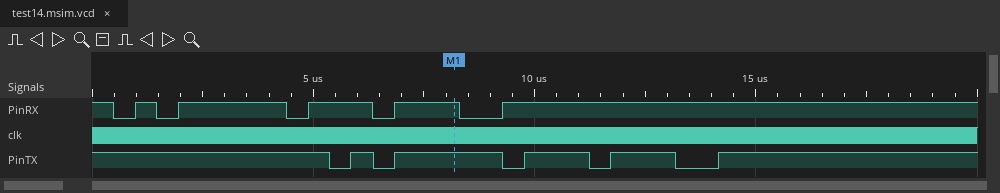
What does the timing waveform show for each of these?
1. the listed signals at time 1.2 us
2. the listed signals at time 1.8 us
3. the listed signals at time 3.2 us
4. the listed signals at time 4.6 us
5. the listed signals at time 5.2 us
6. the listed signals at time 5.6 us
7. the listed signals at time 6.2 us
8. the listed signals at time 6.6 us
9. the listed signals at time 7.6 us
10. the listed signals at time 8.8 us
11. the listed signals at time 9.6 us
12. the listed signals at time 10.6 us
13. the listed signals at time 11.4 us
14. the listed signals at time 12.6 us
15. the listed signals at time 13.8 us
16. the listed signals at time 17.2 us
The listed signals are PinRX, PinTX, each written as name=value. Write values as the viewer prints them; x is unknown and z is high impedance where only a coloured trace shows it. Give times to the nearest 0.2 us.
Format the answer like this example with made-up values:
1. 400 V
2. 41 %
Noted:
1. PinRX=1, PinTX=1
2. PinRX=0, PinTX=1
3. PinRX=1, PinTX=1
4. PinRX=0, PinTX=1
5. PinRX=1, PinTX=1
6. PinRX=1, PinTX=0
7. PinRX=1, PinTX=1
8. PinRX=0, PinTX=0
9. PinRX=1, PinTX=1
10. PinRX=0, PinTX=1
11. PinRX=1, PinTX=0
12. PinRX=1, PinTX=1
13. PinRX=1, PinTX=0
14. PinRX=1, PinTX=1
15. PinRX=1, PinTX=0
16. PinRX=1, PinTX=1
